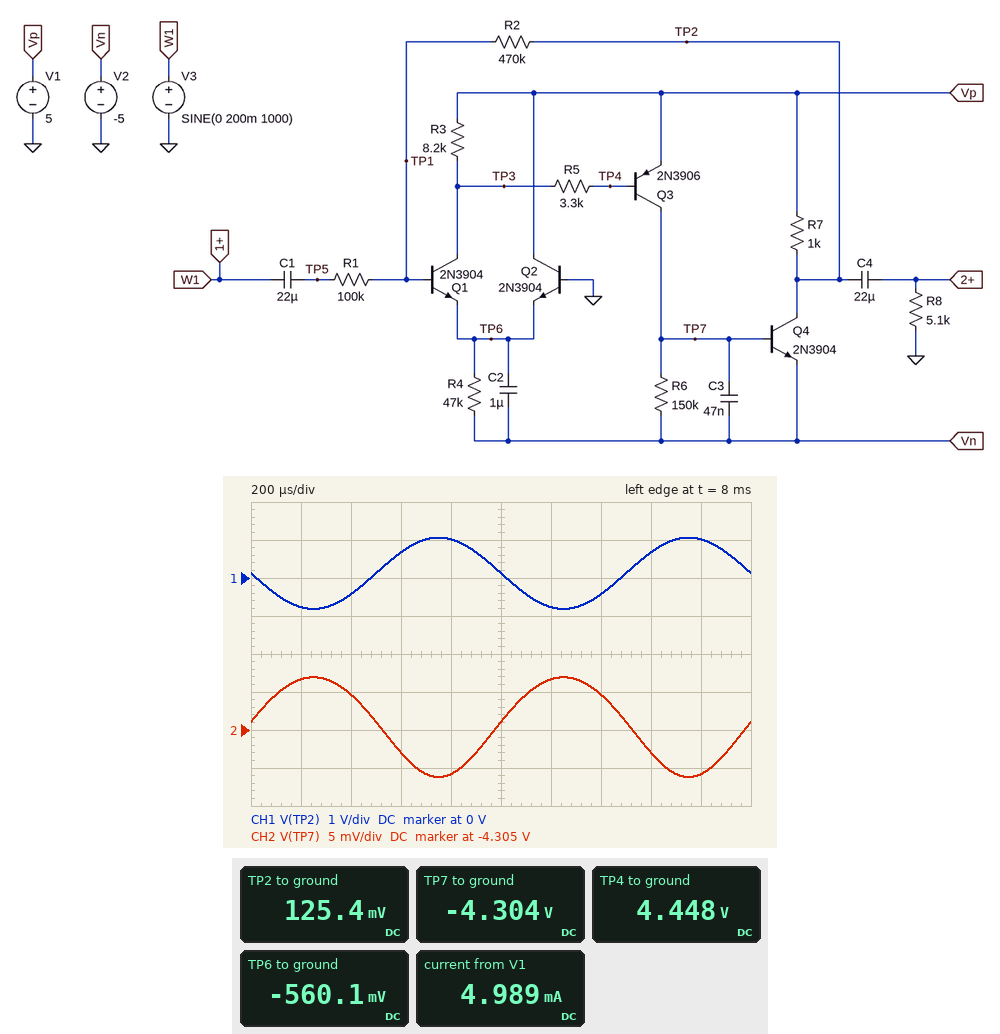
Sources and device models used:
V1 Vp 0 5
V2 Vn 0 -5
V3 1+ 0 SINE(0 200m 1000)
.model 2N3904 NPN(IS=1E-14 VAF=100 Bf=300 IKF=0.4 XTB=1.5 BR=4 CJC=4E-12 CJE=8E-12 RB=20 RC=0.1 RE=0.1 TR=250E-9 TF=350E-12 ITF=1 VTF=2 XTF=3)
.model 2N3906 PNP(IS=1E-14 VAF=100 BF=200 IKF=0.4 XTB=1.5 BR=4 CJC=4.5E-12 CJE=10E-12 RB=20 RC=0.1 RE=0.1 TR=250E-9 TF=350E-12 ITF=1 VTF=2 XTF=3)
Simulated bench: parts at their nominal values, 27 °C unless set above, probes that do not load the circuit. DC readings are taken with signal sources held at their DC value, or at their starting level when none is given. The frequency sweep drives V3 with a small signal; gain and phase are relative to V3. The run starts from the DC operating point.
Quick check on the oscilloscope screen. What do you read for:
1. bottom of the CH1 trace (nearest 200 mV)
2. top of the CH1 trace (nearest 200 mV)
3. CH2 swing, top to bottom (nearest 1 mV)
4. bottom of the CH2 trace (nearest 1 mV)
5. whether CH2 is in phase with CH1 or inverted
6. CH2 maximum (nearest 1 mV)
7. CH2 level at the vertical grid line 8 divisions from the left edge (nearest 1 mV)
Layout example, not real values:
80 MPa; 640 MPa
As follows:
-800 mV; 1.0 V; 13 mV; -4.311 V; inverted; -4.298 V; -4.308 V
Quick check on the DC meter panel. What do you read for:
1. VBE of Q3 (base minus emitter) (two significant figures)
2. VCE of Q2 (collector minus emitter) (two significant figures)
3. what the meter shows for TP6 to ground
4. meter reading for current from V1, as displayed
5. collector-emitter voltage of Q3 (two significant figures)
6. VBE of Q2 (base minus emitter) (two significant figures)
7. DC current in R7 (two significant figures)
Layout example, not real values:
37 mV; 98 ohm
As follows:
-550 mV; 5.6 V; -560.1 mV; 4.989 mA; -9.3 V; 560 mV; 4.9 mA
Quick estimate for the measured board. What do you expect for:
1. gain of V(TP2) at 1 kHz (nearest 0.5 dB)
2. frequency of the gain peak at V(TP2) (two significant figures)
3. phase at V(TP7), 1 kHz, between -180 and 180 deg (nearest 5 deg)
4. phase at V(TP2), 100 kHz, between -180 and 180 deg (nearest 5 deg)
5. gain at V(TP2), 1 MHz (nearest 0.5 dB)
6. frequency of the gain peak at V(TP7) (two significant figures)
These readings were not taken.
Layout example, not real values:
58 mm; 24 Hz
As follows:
13.5 dB; 210 kHz; 0 deg; 170 deg; -14.5 dB; 210 kHz
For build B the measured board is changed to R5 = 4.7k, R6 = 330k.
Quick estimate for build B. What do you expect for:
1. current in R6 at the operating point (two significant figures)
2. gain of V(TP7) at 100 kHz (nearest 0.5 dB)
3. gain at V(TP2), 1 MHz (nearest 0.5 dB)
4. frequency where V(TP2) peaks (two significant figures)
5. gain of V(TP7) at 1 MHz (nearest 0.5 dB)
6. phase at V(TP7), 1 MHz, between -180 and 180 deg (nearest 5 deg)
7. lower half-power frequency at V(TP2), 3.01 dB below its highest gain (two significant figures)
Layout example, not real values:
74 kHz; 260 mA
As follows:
2.1 µA; -27.0 dB; -16.5 dB; 190 kHz; -59.5 dB; 145 deg; 180 kHz
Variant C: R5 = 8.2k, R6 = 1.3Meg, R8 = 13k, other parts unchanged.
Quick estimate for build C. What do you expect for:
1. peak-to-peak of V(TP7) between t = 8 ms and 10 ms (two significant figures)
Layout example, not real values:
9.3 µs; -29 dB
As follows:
12 mV
